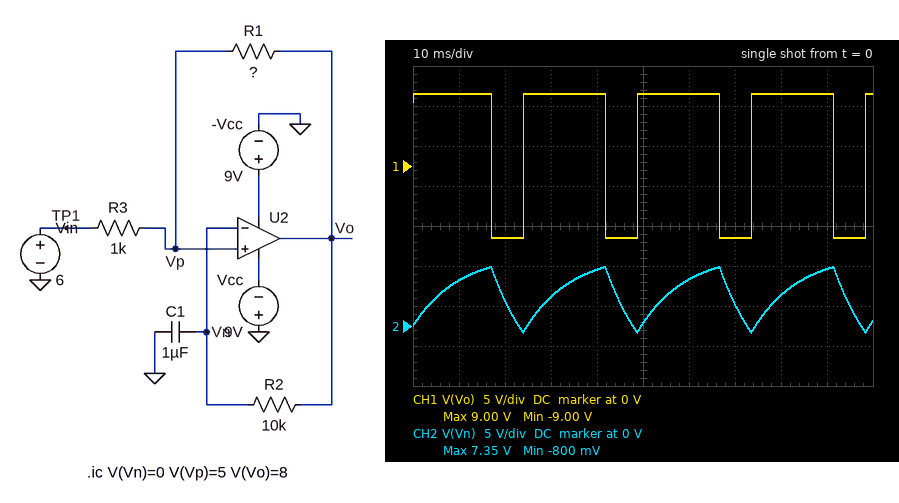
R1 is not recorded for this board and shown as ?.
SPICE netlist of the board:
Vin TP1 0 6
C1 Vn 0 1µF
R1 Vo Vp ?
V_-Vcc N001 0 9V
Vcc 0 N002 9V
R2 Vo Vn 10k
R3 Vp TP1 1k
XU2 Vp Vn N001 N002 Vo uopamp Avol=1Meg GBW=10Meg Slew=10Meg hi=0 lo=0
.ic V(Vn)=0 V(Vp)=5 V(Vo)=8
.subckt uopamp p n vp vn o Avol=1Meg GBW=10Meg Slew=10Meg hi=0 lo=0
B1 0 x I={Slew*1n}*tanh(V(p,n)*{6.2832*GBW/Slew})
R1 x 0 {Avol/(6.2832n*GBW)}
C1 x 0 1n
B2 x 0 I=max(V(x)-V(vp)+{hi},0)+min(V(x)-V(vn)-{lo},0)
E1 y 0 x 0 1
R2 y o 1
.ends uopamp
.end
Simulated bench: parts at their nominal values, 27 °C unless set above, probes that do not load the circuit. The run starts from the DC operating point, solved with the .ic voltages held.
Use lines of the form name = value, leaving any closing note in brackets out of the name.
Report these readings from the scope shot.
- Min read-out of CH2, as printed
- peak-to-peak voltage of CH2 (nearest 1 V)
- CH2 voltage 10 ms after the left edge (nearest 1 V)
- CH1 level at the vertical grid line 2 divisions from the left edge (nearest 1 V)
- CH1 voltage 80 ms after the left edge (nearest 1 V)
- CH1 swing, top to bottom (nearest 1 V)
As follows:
Min read-out of CH2, as printed = -800 mV
peak-to-peak voltage of CH2 = 8 V
CH2 voltage 10 ms after the left edge = 6 V
CH1 level at the vertical grid line 2 divisions from the left edge = -9 V
CH1 voltage 80 ms after the left edge = 9 V
CH1 swing, top to bottom = 18 V
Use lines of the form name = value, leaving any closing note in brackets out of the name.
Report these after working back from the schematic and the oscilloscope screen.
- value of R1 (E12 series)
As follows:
value of R1 = 1.2 kΩ
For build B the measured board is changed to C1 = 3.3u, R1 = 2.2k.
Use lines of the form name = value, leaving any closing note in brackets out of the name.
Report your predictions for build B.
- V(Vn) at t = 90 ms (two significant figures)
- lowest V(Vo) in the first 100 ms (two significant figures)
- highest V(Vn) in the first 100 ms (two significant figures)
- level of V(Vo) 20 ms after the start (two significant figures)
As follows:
V(Vn) at t = 90 ms = 5.6 V
lowest V(Vo) in the first 100 ms = -9.0 V
highest V(Vn) in the first 100 ms = 6.9 V
level of V(Vo) 20 ms after the start = 9.0 V
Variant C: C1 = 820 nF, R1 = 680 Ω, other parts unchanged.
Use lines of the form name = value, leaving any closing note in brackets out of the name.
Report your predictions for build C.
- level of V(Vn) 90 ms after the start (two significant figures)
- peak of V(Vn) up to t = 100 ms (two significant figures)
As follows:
level of V(Vn) 90 ms after the start = 6.0 V
peak of V(Vn) up to t = 100 ms = 7.8 V
